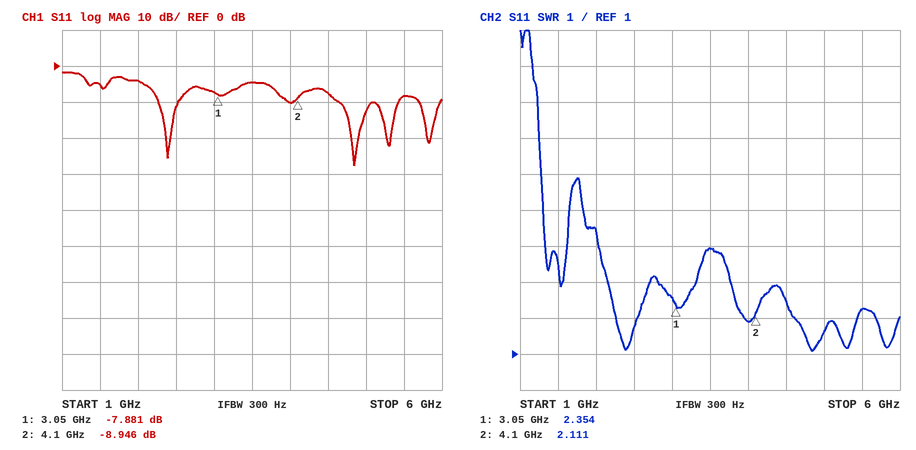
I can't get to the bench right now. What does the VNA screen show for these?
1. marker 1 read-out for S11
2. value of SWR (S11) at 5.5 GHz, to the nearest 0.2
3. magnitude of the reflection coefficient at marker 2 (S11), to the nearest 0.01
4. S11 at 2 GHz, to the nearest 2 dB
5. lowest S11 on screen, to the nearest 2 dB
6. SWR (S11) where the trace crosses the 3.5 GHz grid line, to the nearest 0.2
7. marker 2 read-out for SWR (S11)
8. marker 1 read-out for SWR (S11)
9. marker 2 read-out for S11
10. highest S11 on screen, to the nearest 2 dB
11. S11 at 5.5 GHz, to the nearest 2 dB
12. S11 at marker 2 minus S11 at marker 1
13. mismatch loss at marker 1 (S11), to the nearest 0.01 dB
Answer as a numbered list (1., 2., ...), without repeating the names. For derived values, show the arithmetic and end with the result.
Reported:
1. -7.881 dB
2. 2.2
3. 10^(-8.946/20) ≈ 0.36
4. -4 dB
5. -28 dB
6. 4.0
7. 2.111
8. 2.354
9. -8.946 dB
10. -2 dB
11. -8 dB
12. -8.946 − (-7.881) = -1.065 dB
13. −10 log10(1 − 10^(-7.881/10)) ≈ 0.77 dB
